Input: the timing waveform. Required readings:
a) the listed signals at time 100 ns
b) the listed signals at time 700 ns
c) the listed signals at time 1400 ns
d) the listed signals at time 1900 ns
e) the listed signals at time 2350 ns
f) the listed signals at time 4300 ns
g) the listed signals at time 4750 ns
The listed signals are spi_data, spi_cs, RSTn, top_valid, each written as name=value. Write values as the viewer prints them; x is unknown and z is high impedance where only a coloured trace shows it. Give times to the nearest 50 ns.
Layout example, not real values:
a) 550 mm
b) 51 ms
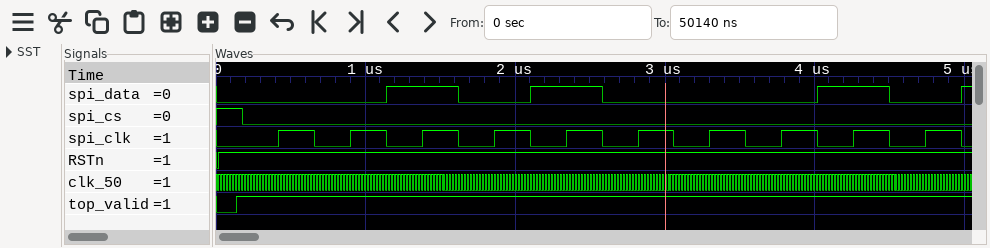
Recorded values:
a) spi_data=0, spi_cs=1, RSTn=1, top_valid=0
b) spi_data=0, spi_cs=0, RSTn=1, top_valid=1
c) spi_data=1, spi_cs=0, RSTn=1, top_valid=1
d) spi_data=0, spi_cs=0, RSTn=1, top_valid=1
e) spi_data=1, spi_cs=0, RSTn=1, top_valid=1
f) spi_data=1, spi_cs=0, RSTn=1, top_valid=1
g) spi_data=0, spi_cs=0, RSTn=1, top_valid=1
